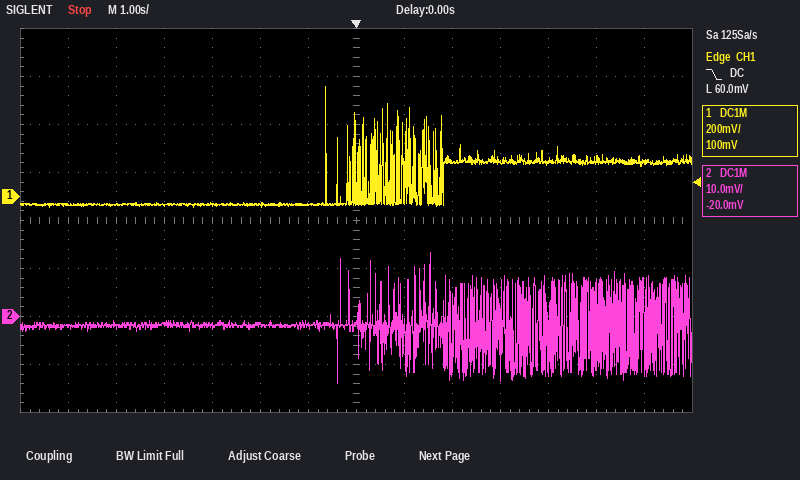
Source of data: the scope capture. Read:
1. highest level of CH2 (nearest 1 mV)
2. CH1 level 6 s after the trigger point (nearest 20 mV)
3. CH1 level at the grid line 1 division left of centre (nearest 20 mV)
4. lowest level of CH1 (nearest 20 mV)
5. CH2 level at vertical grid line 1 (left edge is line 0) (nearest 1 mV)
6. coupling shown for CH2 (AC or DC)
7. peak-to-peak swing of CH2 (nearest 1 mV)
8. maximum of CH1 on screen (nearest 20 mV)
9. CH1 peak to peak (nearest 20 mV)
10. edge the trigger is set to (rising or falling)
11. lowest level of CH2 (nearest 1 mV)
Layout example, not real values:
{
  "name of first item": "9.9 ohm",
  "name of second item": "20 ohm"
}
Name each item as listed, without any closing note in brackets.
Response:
{
  "highest level of CH2": "13 mV",
  "CH1 level 6 s after the trigger point": "140 mV",
  "CH1 level at the grid line 1 division left of centre": "-40 mV",
  "lowest level of CH1": "-40 mV",
  "CH2 level at vertical grid line 1 (left edge is line 0)": "-2 mV",
  "coupling shown for CH2": "DC",
  "peak-to-peak swing of CH2": "27 mV",
  "maximum of CH1 on screen": "460 mV",
  "CH1 peak to peak": "500 mV",
  "edge the trigger is set to": "falling",
  "lowest level of CH2": "-14 mV"
}
